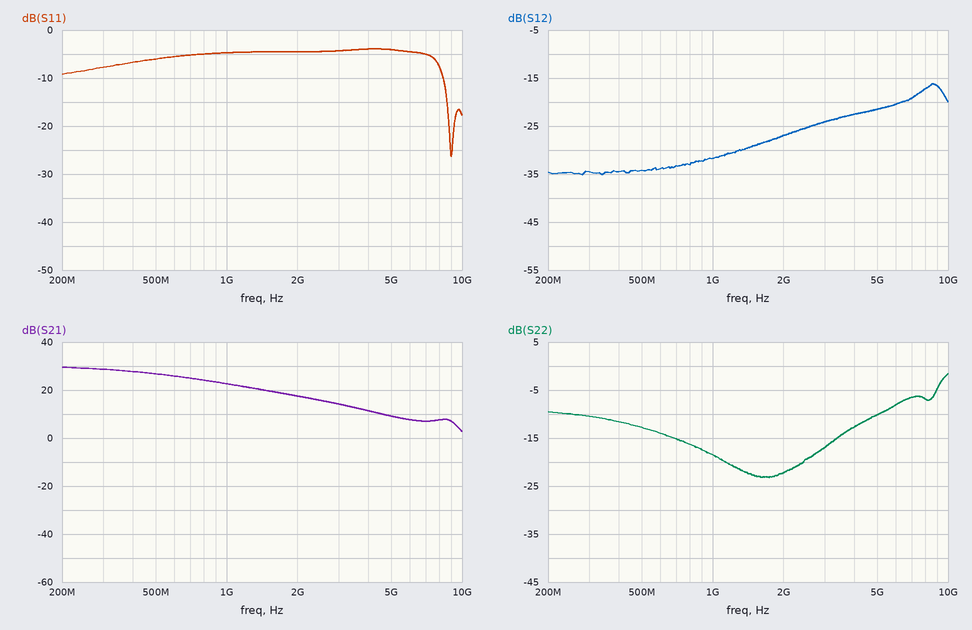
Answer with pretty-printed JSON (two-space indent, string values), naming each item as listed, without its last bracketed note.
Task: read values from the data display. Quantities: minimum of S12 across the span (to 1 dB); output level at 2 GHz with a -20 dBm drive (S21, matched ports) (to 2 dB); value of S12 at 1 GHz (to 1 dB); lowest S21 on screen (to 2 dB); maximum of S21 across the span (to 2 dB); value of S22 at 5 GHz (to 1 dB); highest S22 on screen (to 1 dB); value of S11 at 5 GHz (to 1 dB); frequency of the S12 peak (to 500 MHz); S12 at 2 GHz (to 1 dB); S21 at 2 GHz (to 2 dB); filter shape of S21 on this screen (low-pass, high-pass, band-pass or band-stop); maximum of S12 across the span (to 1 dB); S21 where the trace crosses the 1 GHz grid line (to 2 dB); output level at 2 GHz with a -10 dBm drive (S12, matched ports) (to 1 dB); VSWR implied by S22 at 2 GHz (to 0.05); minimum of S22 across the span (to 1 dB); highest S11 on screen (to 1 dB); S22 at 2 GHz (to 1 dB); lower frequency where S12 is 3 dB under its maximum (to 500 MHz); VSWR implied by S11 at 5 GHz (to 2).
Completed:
{
  "minimum of S12 across the span": "-35 dB",
  "output level at 2 GHz with a -20 dBm drive (S21, matched ports)": "-2 dBm",
  "value of S12 at 1 GHz": "-32 dB",
  "lowest S21 on screen": "2 dB",
  "maximum of S21 across the span": "30 dB",
  "value of S22 at 5 GHz": "-10 dB",
  "highest S22 on screen": "-2 dB",
  "value of S11 at 5 GHz": "-4 dB",
  "frequency of the S12 peak": "8.5 GHz",
  "S12 at 2 GHz": "-27 dB",
  "S21 at 2 GHz": "18 dB",
  "filter shape of S21 on this screen": "low-pass",
  "maximum of S12 across the span": "-16 dB",
  "S21 where the trace crosses the 1 GHz grid line": "22 dB",
  "output level at 2 GHz with a -10 dBm drive (S12, matched ports)": "-37 dBm",
  "VSWR implied by S22 at 2 GHz": "1.15",
  "minimum of S22 across the span": "-23 dB",
  "highest S11 on screen": "-4 dB",
  "S22 at 2 GHz": "-22 dB",
  "lower frequency where S12 is 3 dB under its maximum": "7.0 GHz",
  "VSWR implied by S11 at 5 GHz": "4"
}
